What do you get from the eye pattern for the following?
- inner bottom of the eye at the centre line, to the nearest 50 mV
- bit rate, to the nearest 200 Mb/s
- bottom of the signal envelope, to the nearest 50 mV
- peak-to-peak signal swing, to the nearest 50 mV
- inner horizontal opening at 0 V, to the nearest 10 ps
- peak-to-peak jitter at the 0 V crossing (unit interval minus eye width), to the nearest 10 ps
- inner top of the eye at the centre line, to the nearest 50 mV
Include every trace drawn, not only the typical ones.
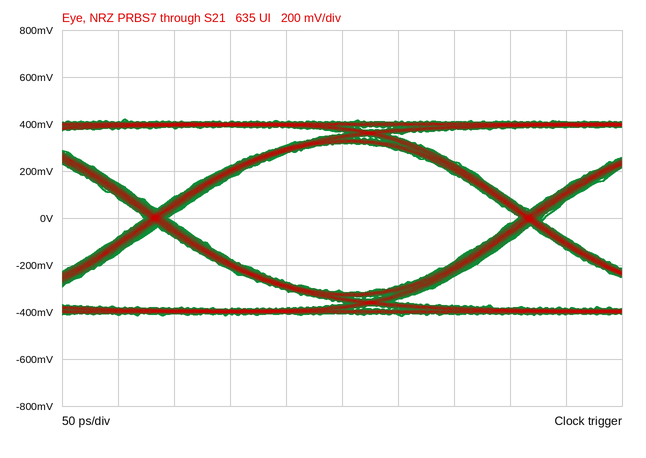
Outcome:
-300 mV
3.0 Gb/s
-400 mV
850 mV
310 ps
20 ps
300 mV
